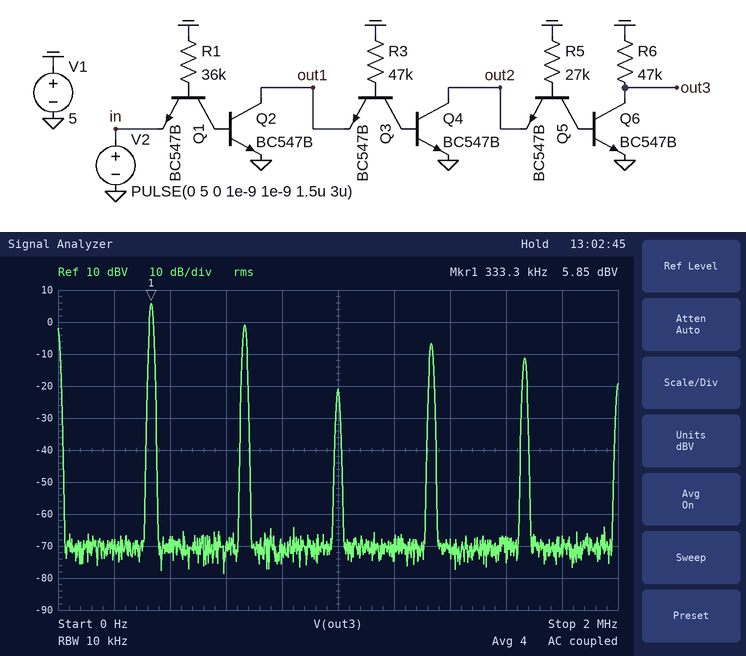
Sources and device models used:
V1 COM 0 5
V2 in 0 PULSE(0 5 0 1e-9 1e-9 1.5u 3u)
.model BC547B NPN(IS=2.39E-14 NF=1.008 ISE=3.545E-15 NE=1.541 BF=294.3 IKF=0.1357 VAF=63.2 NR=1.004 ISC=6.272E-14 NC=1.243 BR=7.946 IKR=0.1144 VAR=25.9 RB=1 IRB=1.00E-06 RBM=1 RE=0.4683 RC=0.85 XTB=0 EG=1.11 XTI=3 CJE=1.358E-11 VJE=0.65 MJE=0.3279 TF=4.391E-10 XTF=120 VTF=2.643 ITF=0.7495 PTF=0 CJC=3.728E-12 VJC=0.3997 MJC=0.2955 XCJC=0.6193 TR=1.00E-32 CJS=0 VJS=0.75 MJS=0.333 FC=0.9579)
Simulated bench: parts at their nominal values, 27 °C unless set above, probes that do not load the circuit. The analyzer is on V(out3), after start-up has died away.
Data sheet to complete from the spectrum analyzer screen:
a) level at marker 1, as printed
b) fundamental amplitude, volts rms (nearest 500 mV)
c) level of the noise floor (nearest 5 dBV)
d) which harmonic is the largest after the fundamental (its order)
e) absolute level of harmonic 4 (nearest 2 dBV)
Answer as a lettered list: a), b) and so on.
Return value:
a) 5.85 dBV
b) 2.0 V
c) -70 dBV
d) 2
e) -6 dBV
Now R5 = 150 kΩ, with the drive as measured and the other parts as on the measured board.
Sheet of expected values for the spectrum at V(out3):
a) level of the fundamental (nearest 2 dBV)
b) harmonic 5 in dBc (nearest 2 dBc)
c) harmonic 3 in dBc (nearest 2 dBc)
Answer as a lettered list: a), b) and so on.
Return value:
a) 6 dBV
b) -24 dBc
c) -16 dBc
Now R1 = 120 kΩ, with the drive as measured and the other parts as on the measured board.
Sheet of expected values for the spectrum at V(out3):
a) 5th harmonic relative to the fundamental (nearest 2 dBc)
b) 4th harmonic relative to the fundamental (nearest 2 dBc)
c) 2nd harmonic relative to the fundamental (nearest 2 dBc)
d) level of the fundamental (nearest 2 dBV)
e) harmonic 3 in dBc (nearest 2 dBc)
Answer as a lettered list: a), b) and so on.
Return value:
a) -14 dBc
b) -8 dBc
c) -2 dBc
d) 0 dBV
e) -4 dBc
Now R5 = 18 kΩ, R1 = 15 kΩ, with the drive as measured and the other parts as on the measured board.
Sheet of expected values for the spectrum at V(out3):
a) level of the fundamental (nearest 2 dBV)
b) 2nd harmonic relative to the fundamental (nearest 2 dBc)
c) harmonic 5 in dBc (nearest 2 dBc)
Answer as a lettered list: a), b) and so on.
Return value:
a) 6 dBV
b) -8 dBc
c) -22 dBc
